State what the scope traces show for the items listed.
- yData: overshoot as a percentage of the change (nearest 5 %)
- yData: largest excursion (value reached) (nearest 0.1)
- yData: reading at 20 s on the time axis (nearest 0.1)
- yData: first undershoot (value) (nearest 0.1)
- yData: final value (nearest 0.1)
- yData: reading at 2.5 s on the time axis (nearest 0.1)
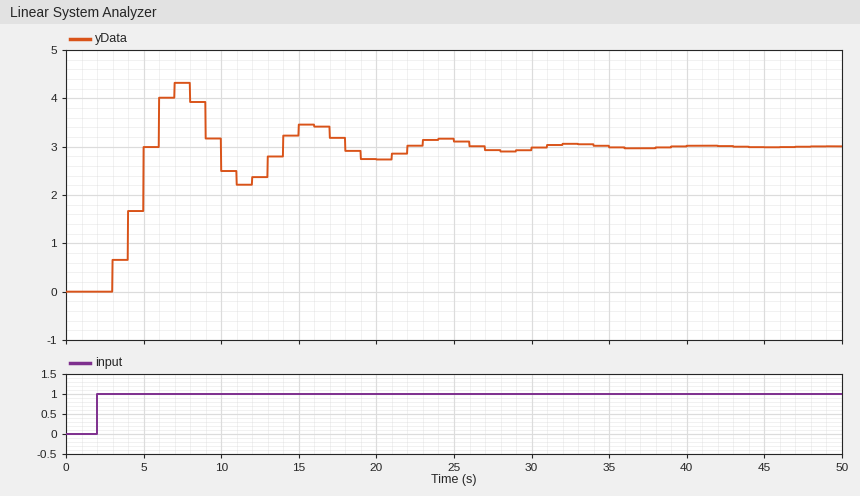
45 %
4.3
2.7
2.2
3.0
0.0
